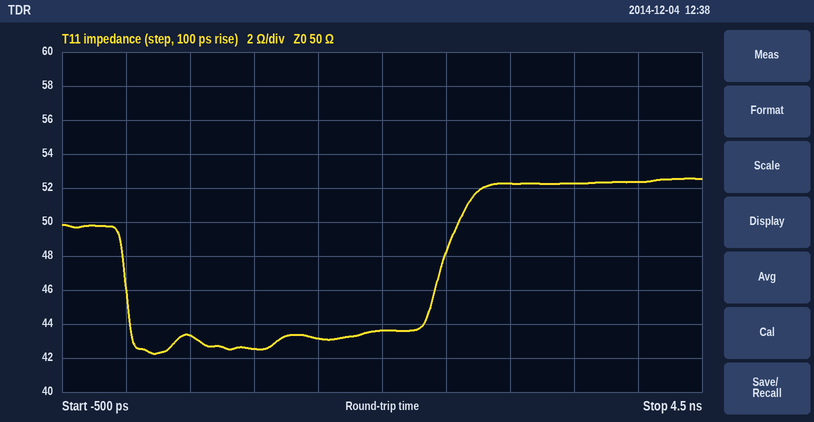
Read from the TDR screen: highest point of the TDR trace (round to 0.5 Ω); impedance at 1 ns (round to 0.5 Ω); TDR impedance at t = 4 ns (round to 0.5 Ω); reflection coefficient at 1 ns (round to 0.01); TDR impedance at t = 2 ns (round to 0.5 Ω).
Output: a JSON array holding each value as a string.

["52.5 Ω", "42.5 Ω", "52.5 Ω", "-0.08", "43.5 Ω"]
